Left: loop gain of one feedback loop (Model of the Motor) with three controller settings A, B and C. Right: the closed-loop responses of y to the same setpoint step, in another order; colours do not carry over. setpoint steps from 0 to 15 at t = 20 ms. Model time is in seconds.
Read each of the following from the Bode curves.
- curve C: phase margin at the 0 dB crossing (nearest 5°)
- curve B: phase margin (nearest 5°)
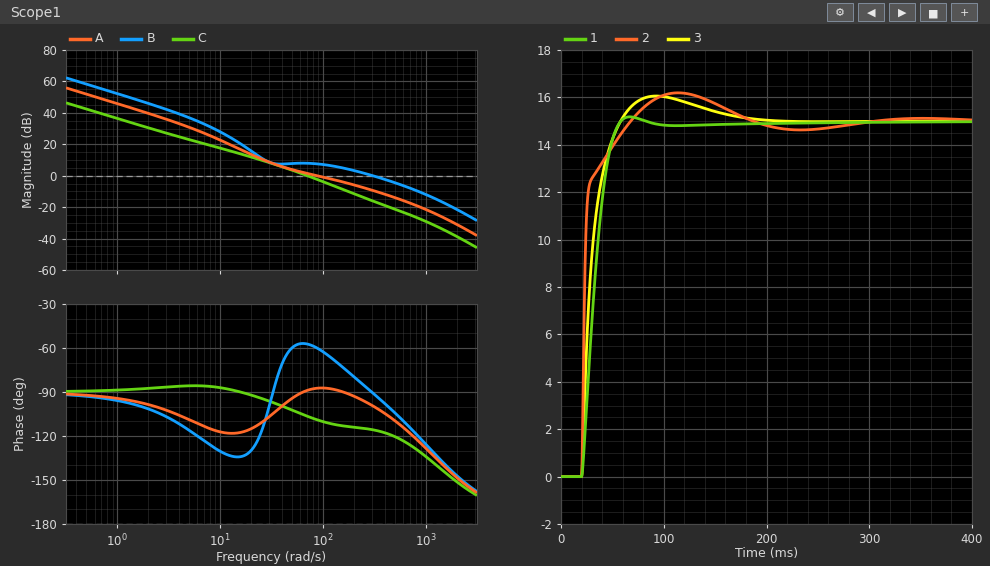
75°
90°
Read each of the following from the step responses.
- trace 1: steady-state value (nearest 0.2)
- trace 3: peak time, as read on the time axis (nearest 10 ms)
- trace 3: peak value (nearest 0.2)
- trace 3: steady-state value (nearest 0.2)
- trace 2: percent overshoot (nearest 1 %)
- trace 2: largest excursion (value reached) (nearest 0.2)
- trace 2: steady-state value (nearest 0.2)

15.0
90 ms
16.0
15.0
8 %
16.2
15.0
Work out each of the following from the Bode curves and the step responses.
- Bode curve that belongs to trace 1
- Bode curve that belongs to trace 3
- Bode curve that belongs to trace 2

C
A
B
